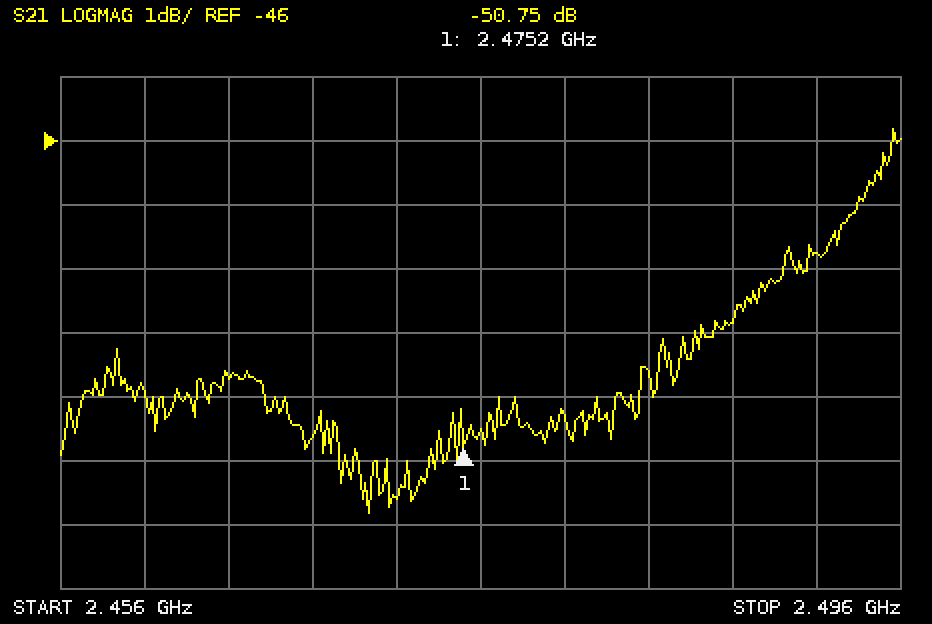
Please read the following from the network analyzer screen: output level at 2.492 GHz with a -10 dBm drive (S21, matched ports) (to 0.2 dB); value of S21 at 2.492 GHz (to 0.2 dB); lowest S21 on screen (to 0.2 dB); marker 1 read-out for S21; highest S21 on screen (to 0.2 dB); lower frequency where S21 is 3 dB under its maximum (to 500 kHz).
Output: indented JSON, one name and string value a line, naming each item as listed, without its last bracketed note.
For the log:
{
  "output level at 2.492 GHz with a -10 dBm drive (S21, matched ports)": "-57.8 dBm",
  "value of S21 at 2.492 GHz": "-47.8 dB",
  "lowest S21 on screen": "-51.8 dB",
  "marker 1 read-out for S21": "-50.75 dB",
  "highest S21 on screen": "-45.8 dB",
  "lower frequency where S21 is 3 dB under its maximum": "2.4880 GHz"
}
